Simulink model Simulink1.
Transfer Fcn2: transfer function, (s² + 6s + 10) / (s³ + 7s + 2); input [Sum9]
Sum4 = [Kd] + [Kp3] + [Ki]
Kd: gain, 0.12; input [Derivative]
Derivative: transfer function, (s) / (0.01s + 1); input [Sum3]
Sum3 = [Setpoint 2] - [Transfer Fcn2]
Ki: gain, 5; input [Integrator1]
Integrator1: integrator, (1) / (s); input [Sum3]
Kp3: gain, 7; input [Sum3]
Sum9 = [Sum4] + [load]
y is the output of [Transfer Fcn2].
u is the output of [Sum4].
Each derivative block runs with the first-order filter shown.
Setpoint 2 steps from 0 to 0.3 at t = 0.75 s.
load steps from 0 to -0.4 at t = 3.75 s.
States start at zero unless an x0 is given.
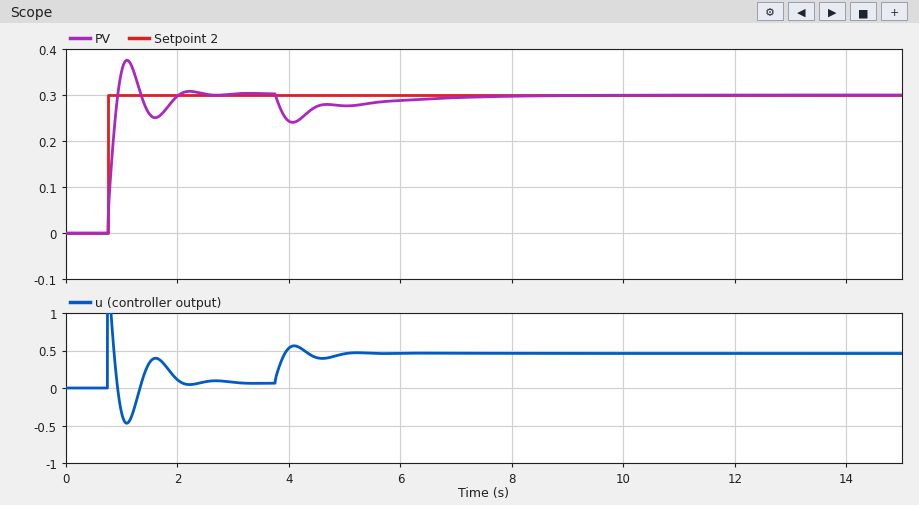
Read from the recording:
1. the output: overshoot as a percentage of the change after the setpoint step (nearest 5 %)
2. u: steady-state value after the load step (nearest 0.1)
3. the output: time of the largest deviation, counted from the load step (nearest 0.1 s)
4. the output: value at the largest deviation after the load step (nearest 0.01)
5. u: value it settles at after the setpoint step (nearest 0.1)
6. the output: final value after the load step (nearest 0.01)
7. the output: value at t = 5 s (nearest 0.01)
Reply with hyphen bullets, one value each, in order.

- 25 %
- 0.5
- 0.3 s
- 0.24
- 0.1
- 0.30
- 0.28
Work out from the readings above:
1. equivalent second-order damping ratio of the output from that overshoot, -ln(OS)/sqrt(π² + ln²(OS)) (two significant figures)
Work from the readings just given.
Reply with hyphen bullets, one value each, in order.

- 0.40
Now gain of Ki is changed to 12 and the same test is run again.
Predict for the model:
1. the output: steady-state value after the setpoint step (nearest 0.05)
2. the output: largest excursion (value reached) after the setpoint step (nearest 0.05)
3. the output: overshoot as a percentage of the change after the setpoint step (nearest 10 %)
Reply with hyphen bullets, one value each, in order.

- 0.30
- 0.40
- 30 %
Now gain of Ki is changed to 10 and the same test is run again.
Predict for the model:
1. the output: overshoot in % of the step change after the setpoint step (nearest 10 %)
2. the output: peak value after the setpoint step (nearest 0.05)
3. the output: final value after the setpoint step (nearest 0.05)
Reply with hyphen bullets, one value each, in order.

- 30 %
- 0.40
- 0.30
